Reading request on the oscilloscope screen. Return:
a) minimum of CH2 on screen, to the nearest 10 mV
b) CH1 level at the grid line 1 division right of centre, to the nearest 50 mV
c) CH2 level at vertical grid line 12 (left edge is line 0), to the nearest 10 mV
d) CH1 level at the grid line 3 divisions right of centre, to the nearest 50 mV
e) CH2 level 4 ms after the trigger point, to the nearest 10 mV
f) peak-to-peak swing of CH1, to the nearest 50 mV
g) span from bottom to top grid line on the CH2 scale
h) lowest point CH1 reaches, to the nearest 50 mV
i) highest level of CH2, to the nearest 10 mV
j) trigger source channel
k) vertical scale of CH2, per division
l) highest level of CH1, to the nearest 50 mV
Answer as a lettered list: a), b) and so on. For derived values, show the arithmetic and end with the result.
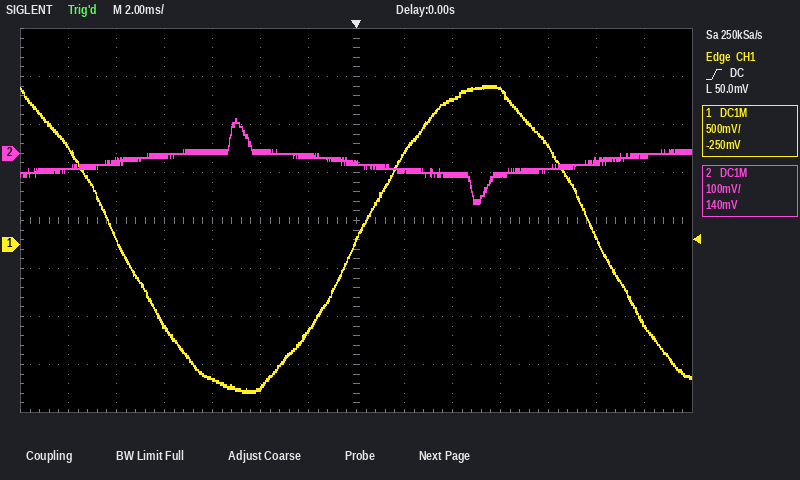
a) -100 mV
b) 950 mV
c) -20 mV
d) 1.60 V
e) -40 mV
f) 1.65 V − (-1.55 V) = 3.20 V
g) 800 mV
h) -1.55 V
i) 70 mV
j) CH1
k) 100 mV
l) 1.65 V
